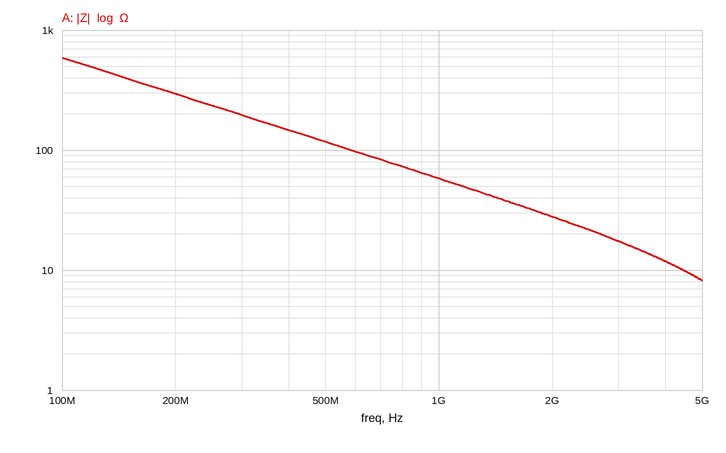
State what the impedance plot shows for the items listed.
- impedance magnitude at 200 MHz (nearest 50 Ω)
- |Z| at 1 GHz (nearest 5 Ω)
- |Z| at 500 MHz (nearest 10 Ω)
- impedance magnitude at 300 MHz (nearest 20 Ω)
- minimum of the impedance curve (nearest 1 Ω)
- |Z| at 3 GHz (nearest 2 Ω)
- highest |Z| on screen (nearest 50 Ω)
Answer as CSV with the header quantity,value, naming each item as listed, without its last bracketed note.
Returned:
quantity,value
impedance magnitude at 200 MHz,300 Ω
|Z| at 1 GHz,60 Ω
|Z| at 500 MHz,120 Ω
impedance magnitude at 300 MHz,200 Ω
minimum of the impedance curve,8 Ω
|Z| at 3 GHz,18 Ω
highest |Z| on screen,600 Ω
